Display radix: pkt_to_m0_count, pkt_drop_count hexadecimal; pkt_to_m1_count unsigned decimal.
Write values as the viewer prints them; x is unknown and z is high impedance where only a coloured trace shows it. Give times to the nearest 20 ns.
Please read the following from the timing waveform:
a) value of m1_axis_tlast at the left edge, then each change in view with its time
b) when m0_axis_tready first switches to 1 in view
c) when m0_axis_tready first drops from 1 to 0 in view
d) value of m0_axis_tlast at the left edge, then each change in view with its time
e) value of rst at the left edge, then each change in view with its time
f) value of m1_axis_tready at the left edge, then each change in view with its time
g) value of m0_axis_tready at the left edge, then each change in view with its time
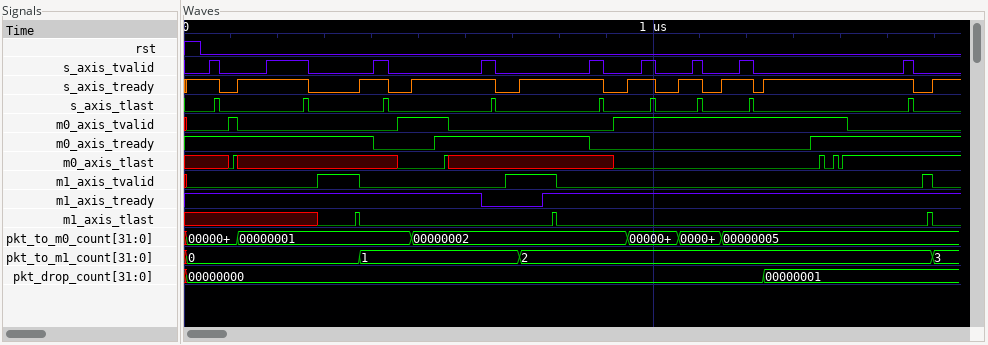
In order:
x, 0 at 280 ns, 1 at 360 ns, 0 at 380 ns, 1 at 780 ns, 0 at 800 ns, 1 at 1580 ns, 0 at 1600 ns
540 ns
400 ns
x, 0 at 100 ns, 1 at 100 ns, x at 120 ns, 0 at 460 ns, 1 at 560 ns, x at 560 ns, 0 at 920 ns, 1 at 1360 ns, 0 at 1360 ns, 1 at 1380 ns, 0 at 1400 ns, 1 at 1400 ns
1, 0 at 40 ns
1, 0 at 640 ns, 1 at 760 ns
1, 0 at 400 ns, 1 at 540 ns, 0 at 860 ns, 1 at 1340 ns
